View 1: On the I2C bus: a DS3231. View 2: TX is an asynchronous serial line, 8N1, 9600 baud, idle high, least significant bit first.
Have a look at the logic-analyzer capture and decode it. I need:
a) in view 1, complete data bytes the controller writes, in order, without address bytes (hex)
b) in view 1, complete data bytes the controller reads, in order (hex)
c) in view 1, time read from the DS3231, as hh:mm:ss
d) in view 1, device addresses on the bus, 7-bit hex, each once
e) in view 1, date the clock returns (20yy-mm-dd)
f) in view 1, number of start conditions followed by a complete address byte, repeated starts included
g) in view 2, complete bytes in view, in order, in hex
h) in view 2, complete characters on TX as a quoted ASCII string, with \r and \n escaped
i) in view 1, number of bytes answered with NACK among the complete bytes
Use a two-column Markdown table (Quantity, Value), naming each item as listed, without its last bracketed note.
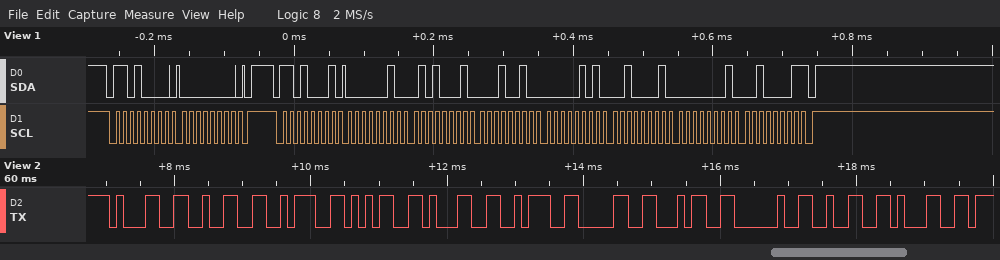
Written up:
| Quantity | Value |
|---|---|
| in view 1, complete data bytes the controller writes, in order, without address bytes | 00 |
| in view 1, complete data bytes the controller reads, in order | 02 51 12 05 21 01 21 |
| in view 1, time read from the DS3231, as hh:mm:ss | 12:51:02 |
| in view 1, device addresses on the bus, 7-bit hex, each once | 0x68 |
| in view 1, date the clock returns | 2021-01-21 |
| in view 1, number of start conditions followed by a complete address byte, repeated starts included | 2 |
| in view 2, complete bytes in view, in order, in hex | 31 32 3A 35 31 3A 30 34 20 32 31 |
| in view 2, complete characters on TX as a quoted ASCII string, with \r and \n escaped | "12:51:04 21" |
| in view 1, number of bytes answered with NACK among the complete bytes | 1 |
